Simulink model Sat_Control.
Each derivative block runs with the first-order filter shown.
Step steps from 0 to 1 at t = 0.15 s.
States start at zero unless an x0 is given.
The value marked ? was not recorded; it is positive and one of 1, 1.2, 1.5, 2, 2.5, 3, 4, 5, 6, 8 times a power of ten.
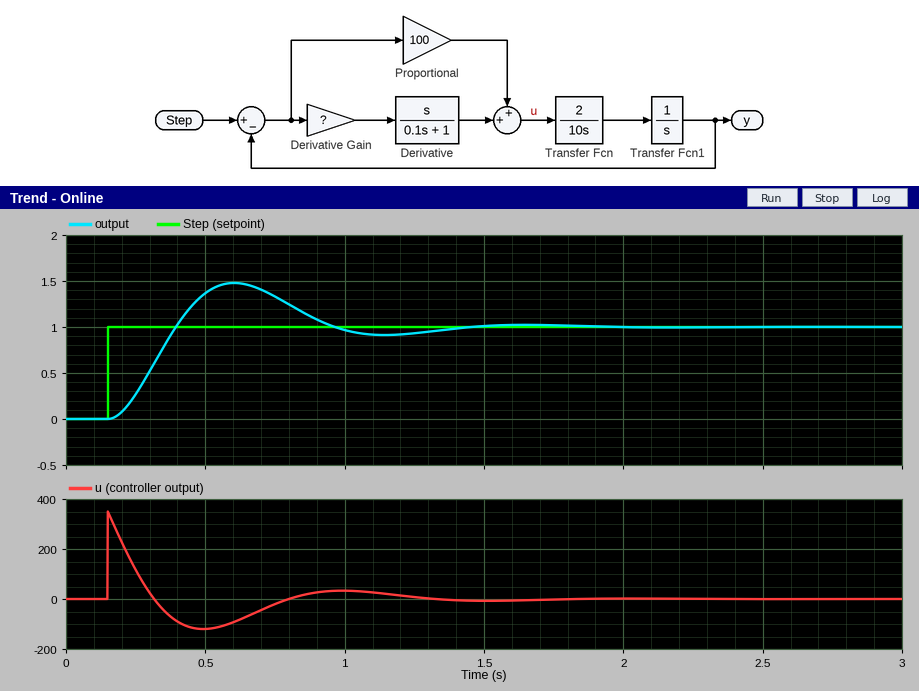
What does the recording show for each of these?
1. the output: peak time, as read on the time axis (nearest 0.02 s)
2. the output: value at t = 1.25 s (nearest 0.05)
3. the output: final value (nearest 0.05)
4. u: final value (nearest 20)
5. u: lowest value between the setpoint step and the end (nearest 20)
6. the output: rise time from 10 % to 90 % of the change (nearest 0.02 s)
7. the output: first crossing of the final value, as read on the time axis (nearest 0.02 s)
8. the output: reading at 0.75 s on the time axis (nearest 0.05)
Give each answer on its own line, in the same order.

0.60 s
0.95
1.00
0
-120
0.16 s
0.40 s
1.35
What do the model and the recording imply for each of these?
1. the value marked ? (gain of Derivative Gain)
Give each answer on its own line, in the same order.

25
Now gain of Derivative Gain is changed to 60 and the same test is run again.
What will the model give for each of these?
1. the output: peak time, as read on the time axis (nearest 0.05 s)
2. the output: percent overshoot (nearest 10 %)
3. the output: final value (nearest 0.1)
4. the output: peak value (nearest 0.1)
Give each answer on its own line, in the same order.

0.45 s
40 %
1.0
1.4
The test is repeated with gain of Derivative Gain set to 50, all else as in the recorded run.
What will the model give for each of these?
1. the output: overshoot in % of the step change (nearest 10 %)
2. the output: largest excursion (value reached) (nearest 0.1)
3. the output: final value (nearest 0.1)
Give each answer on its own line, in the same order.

40 %
1.4
1.0
